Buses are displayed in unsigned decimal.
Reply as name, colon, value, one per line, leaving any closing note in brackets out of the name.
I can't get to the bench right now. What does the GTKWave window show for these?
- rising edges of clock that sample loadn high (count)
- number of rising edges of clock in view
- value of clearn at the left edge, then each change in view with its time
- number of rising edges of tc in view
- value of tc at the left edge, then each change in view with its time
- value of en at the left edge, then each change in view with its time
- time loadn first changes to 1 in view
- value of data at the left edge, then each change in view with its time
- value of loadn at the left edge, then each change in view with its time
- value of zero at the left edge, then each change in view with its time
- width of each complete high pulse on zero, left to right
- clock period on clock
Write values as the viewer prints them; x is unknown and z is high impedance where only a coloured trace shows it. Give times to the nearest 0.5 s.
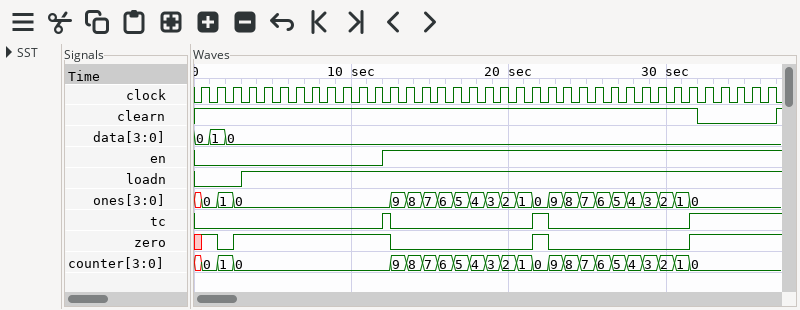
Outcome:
rising edges of clock that sample loadn high: 34
number of rising edges of clock in view: 37
value of clearn at the left edge, then each change in view with its time: 1, 0 at 32 s, 1 at 37 s
number of rising edges of tc in view: 3
value of tc at the left edge, then each change in view with its time: 0, 1 at 12 s, 0 at 12.5 s, 1 at 21.5 s, 0 at 22.5 s, 1 at 31.5 s
value of en at the left edge, then each change in view with its time: 0, 1 at 12 s
time loadn first changes to 1 in view: 3 s
value of data at the left edge, then each change in view with its time: 0, 1 at 1 s, 0 at 2 s
value of loadn at the left edge, then each change in view with its time: 0, 1 at 3 s
value of zero at the left edge, then each change in view with its time: x, 1 at 0.5 s, 0 at 1.5 s, 1 at 2.5 s, 0 at 12.5 s, 1 at 21.5 s, 0 at 22.5 s, 1 at 31.5 s
width of each complete high pulse on zero, left to right: 10 s, 1 s
clock period on clock: 1 s
